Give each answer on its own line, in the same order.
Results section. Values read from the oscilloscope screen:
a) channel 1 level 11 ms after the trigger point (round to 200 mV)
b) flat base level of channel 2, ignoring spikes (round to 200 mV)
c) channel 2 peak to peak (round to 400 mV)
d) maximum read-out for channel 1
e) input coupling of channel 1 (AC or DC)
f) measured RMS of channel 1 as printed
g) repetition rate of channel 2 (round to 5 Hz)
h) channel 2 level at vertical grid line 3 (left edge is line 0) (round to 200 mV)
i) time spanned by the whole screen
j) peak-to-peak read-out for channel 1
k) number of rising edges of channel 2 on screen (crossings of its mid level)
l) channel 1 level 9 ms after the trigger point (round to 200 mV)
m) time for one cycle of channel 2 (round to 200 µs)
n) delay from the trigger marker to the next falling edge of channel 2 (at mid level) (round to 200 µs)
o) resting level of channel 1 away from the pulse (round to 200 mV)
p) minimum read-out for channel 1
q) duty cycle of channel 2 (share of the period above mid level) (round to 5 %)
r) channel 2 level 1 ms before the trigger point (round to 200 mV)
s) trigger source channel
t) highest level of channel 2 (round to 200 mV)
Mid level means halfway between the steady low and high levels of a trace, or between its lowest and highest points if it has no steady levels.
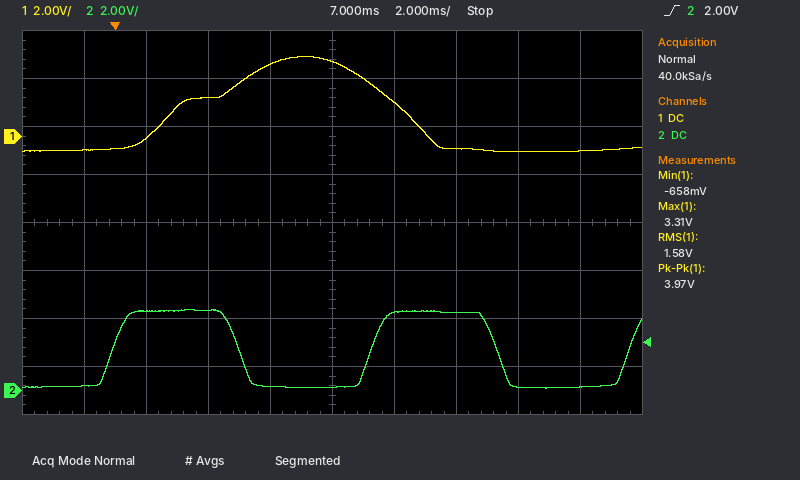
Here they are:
-600 mV
200 mV
3.2 V
3.31 V
DC
1.58 V
120 Hz
3.4 V
20 ms
3.97 V
3
1.4 V
8.4 ms
4.0 ms
-600 mV
-658 mV
50 %
200 mV
channel 2
3.4 V
